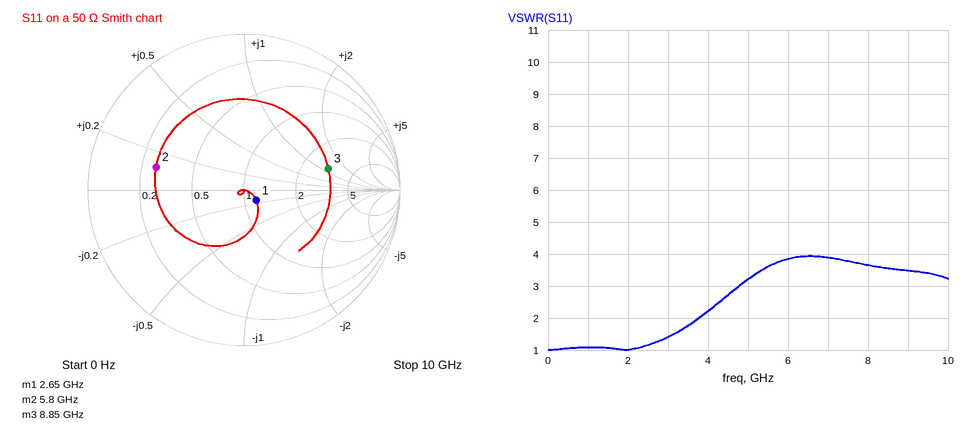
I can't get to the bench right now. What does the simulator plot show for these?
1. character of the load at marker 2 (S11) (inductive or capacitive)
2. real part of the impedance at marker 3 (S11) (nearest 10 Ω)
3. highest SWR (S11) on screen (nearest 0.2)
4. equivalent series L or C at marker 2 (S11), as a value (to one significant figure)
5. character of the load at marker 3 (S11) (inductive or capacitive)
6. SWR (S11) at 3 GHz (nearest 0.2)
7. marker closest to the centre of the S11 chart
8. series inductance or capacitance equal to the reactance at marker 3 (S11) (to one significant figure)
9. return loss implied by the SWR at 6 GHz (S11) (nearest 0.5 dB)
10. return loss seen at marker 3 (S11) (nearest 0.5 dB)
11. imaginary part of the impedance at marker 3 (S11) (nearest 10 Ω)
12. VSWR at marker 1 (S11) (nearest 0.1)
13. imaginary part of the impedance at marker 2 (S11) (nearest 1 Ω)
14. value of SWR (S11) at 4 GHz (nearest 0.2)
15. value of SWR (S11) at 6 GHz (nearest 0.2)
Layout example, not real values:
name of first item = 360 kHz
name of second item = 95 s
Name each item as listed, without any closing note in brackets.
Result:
character of the load at marker 2 (S11) = inductive
real part of the impedance at marker 3 (S11) = 150 Ω
highest SWR (S11) on screen = 4.0
equivalent series L or C at marker 2 (S11), as a value = 200 pH
character of the load at marker 3 (S11) = inductive
SWR (S11) at 3 GHz = 1.4
marker closest to the centre of the S11 chart = marker 1
series inductance or capacitance equal to the reactance at marker 3 (S11) = 1 nH
return loss implied by the SWR at 6 GHz (S11) = 4.5 dB
return loss seen at marker 3 (S11) = 5.0 dB
imaginary part of the impedance at marker 3 (S11) = +60 Ω
VSWR at marker 1 (S11) = 1.2
imaginary part of the impedance at marker 2 (S11) = +6 Ω
value of SWR (S11) at 4 GHz = 2.2
value of SWR (S11) at 6 GHz = 3.8
